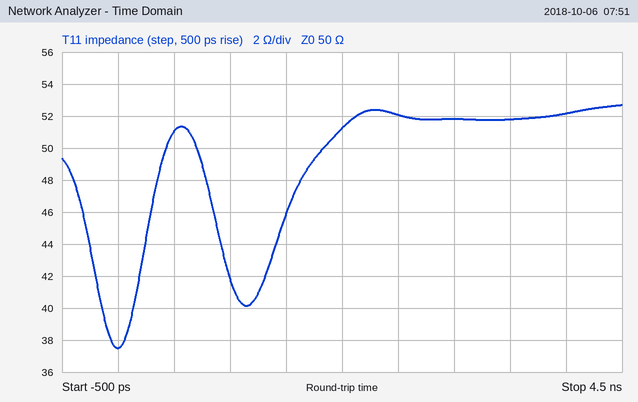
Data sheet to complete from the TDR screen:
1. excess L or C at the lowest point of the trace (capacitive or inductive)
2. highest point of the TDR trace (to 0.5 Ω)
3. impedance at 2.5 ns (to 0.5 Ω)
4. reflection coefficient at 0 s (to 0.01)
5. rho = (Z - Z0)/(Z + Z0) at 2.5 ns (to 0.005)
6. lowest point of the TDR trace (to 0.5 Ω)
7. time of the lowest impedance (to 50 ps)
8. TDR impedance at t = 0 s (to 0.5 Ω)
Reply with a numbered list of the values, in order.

1. capacitive
2. 52.5 Ω
3. 52.0 Ω
4. -0.14
5. +0.020
6. 37.5 Ω
7. 0 ps
8. 37.5 Ω
